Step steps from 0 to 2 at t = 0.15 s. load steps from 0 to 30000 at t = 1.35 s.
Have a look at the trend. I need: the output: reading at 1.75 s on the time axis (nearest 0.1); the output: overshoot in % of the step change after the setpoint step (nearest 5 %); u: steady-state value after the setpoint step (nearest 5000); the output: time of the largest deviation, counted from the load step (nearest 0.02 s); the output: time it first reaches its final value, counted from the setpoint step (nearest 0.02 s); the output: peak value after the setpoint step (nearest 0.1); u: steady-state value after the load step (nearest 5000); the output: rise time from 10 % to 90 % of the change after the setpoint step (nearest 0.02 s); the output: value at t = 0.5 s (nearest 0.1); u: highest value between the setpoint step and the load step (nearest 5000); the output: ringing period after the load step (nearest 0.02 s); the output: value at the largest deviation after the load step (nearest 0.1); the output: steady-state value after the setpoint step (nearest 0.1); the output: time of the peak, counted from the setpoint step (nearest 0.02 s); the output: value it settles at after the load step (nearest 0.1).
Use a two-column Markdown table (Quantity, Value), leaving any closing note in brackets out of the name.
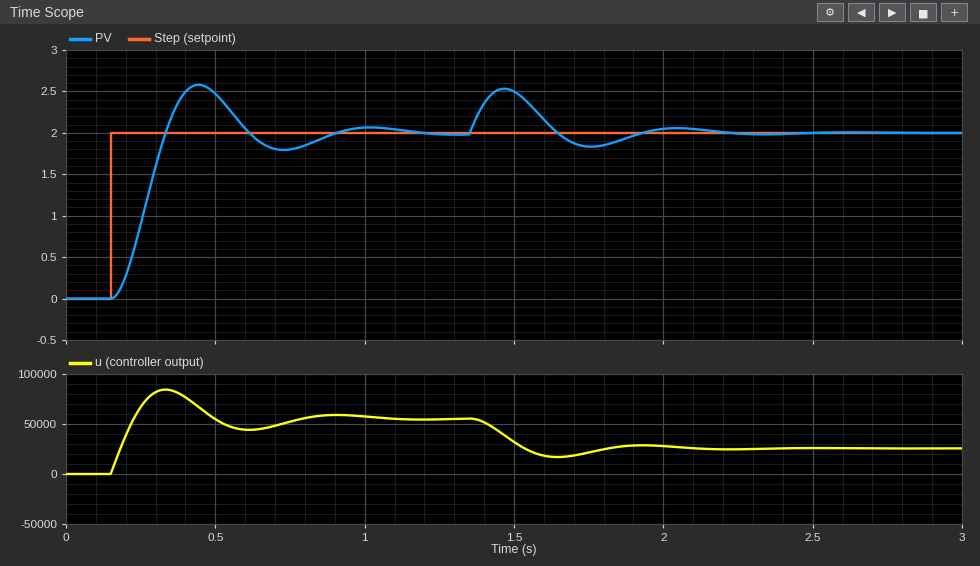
| Quantity | Value |
|---|---|
| the output: reading at 1.75 s on the time axis | 1.8 |
| the output: overshoot in % of the step change after the setpoint step | 30 % |
| u: steady-state value after the setpoint step | 55000 |
| the output: time of the largest deviation, counted from the load step | 0.12 s |
| the output: time it first reaches its final value, counted from the setpoint step | 0.18 s |
| the output: peak value after the setpoint step | 2.6 |
| u: steady-state value after the load step | 25000 |
| the output: rise time from 10 % to 90 % of the change after the setpoint step | 0.12 s |
| the output: value at t = 0.5 s | 2.5 |
| u: highest value between the setpoint step and the load step | 85000 |
| the output: ringing period after the load step | 0.58 s |
| the output: value at the largest deviation after the load step | 2.5 |
| the output: steady-state value after the setpoint step | 2.0 |
| the output: time of the peak, counted from the setpoint step | 0.30 s |
| the output: value it settles at after the load step | 2.0 |
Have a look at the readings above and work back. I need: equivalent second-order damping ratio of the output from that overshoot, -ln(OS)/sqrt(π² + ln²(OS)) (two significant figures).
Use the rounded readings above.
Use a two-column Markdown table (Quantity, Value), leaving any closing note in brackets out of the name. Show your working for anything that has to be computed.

| Quantity | Value |
|---|---|
| equivalent second-order damping ratio of the output from that overshoot, -ln(OS)/sqrt(π² + ln²(OS)) | ln(0.3) = -1.204; 1.204 / sqrt(9.870 + 1.450) = 0.36 |
